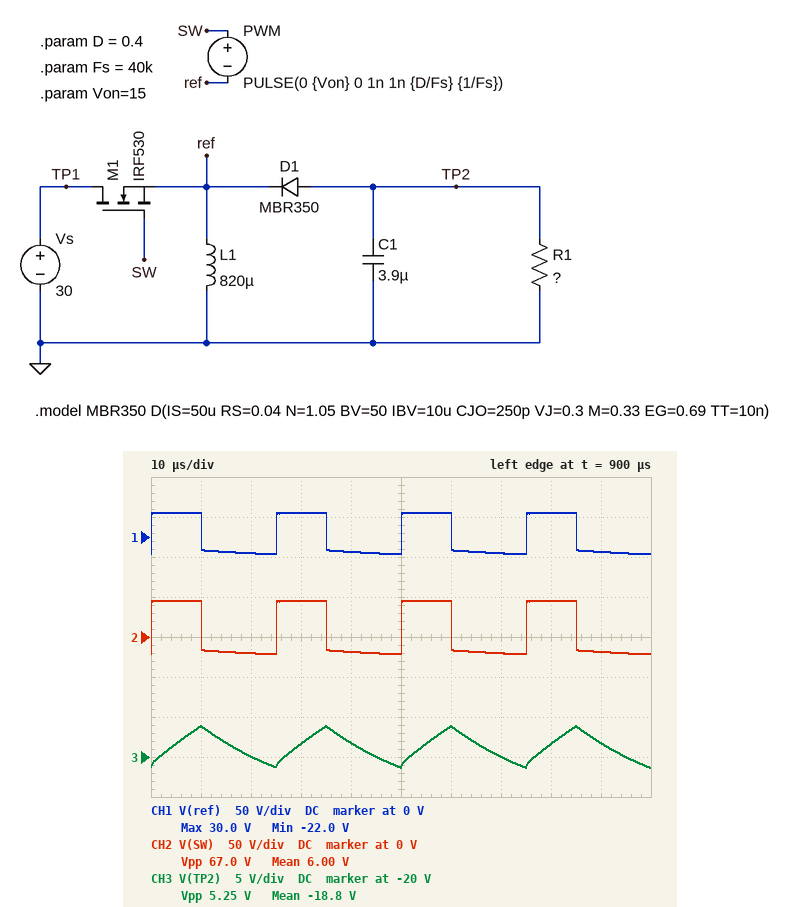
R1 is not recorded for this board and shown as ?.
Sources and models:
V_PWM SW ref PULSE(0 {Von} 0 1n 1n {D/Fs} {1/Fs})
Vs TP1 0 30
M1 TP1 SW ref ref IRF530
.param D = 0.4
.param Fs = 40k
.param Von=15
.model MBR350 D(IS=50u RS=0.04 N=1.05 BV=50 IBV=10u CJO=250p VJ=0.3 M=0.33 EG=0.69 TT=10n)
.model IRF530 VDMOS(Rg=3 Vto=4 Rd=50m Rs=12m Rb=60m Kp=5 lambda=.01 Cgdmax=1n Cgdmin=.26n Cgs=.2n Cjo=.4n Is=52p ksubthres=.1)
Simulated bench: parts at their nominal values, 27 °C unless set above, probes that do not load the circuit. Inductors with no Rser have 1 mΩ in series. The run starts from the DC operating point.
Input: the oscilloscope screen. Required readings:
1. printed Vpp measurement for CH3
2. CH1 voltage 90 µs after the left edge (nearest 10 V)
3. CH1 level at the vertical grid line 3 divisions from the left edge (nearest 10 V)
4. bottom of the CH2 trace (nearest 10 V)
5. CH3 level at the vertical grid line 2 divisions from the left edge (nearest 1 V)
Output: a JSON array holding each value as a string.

["5.25 V", "-20 V", "30 V", "-20 V", "-20 V"]
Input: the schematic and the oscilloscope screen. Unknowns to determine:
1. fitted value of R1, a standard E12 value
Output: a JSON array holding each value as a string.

["10 Ω"]
